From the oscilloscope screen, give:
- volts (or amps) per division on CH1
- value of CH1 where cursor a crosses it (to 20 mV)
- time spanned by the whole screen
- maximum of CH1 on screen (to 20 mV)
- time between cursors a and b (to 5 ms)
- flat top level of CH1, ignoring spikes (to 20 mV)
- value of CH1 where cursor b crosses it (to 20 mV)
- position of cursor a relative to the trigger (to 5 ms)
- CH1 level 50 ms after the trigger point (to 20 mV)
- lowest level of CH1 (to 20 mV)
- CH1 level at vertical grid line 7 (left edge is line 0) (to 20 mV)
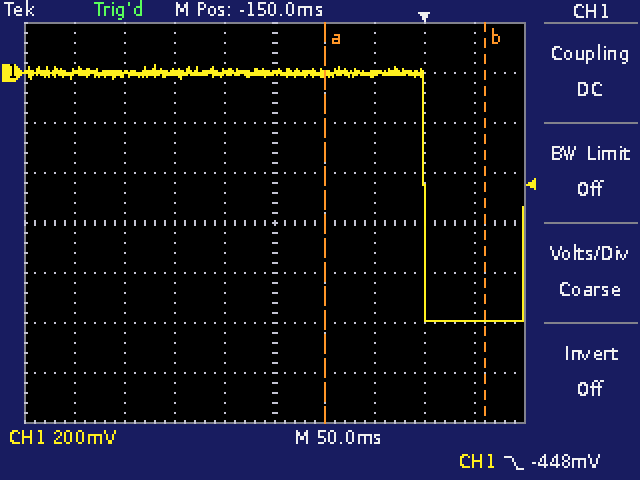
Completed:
200 mV
0 mV
500 ms
40 mV
160 ms
0 mV
-1.00 V
-100 ms
-1.00 V
-1.00 V
0 mV
